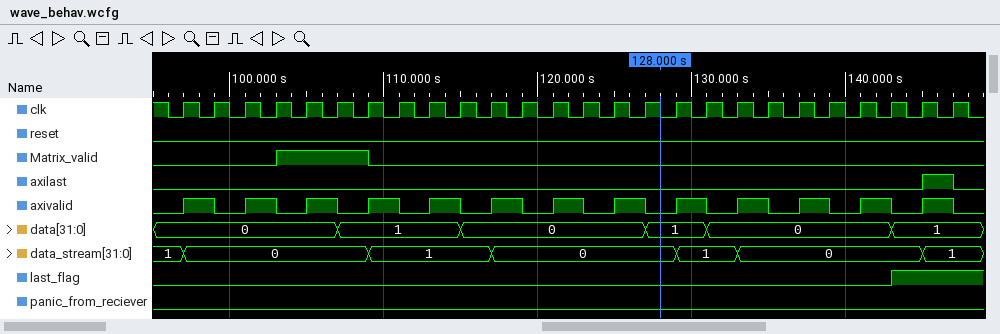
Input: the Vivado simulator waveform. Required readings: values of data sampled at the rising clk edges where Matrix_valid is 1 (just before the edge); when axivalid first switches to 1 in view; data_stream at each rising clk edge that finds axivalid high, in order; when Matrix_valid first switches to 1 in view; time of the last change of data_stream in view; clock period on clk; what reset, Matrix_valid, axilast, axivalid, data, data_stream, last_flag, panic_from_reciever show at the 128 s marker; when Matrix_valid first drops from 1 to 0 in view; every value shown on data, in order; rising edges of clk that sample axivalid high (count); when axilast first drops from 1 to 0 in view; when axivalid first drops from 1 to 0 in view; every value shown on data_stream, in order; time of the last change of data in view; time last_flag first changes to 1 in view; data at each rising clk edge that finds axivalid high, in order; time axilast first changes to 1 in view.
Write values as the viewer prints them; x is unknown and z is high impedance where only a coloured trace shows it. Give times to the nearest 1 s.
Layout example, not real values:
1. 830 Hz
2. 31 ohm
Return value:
1. 0, 0, 1
2. 97 s
3. 0, 0, 0, 1, 1, 0, 0, 0, 1, 0, 0, 0, 1
4. 103 s
5. 145 s
6. 2 s
7. reset=0, Matrix_valid=0, axilast=0, axivalid=0, data=1, data_stream=0, last_flag=0, panic_from_reciever=0
8. 109 s
9. 0, 1, 0, 1, 0, 1
10. 13
11. 147 s
12. 99 s
13. 1, 0, 1, 0, 1, 0, 1
14. 143 s
15. 143 s
16. 0, 0, 0, 1, 1, 0, 0, 0, 1, 0, 0, 0, 1
17. 145 s
